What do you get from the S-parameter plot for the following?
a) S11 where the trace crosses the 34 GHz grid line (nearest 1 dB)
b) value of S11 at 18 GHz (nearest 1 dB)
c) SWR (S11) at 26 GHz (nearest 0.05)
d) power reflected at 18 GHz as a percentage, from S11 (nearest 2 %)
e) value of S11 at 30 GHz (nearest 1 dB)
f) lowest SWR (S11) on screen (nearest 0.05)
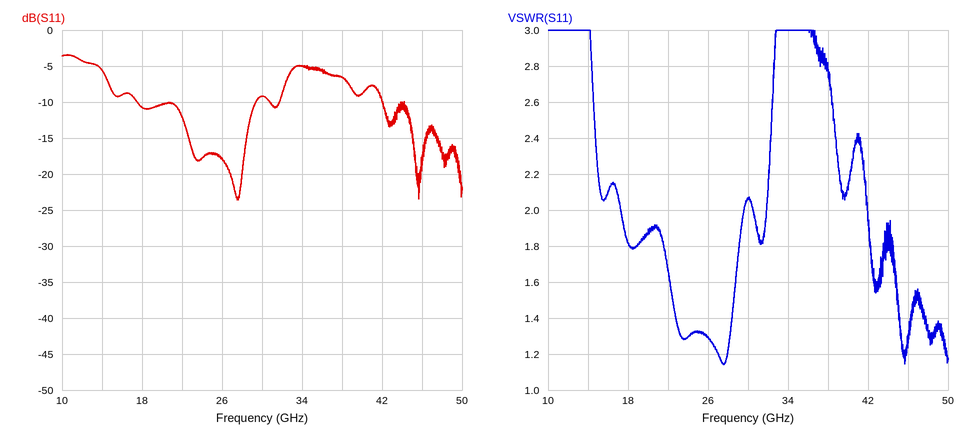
-5 dB
-11 dB
1.30
8 %
-9 dB
1.15
